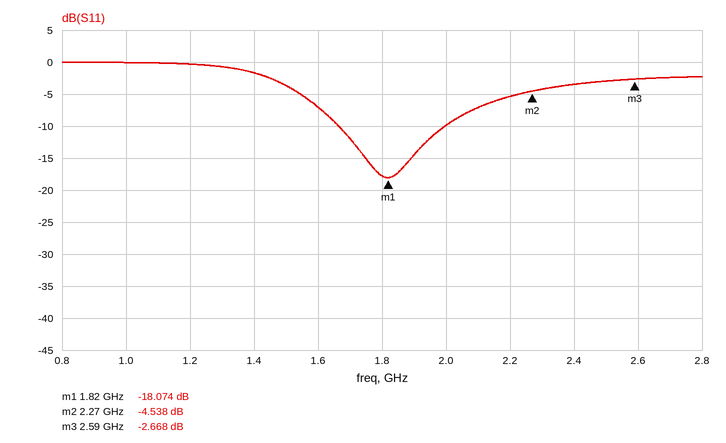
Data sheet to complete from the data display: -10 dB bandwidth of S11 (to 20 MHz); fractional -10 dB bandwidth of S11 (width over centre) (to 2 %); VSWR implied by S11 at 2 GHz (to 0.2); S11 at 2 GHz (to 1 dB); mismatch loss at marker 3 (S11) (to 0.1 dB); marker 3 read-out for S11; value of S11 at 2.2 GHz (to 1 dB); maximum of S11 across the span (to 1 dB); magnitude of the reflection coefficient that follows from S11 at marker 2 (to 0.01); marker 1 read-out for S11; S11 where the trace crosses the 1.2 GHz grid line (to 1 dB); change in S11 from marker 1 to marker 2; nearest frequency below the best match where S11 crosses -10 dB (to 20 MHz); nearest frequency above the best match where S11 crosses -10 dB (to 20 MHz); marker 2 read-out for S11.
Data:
340 MHz
18 %
2.0
-10 dB
3.4 dB
-2.668 dB
-5 dB
0 dB
0.59
-18.074 dB
0 dB
13.536 dB
1.66 GHz
2.00 GHz
-4.538 dB
